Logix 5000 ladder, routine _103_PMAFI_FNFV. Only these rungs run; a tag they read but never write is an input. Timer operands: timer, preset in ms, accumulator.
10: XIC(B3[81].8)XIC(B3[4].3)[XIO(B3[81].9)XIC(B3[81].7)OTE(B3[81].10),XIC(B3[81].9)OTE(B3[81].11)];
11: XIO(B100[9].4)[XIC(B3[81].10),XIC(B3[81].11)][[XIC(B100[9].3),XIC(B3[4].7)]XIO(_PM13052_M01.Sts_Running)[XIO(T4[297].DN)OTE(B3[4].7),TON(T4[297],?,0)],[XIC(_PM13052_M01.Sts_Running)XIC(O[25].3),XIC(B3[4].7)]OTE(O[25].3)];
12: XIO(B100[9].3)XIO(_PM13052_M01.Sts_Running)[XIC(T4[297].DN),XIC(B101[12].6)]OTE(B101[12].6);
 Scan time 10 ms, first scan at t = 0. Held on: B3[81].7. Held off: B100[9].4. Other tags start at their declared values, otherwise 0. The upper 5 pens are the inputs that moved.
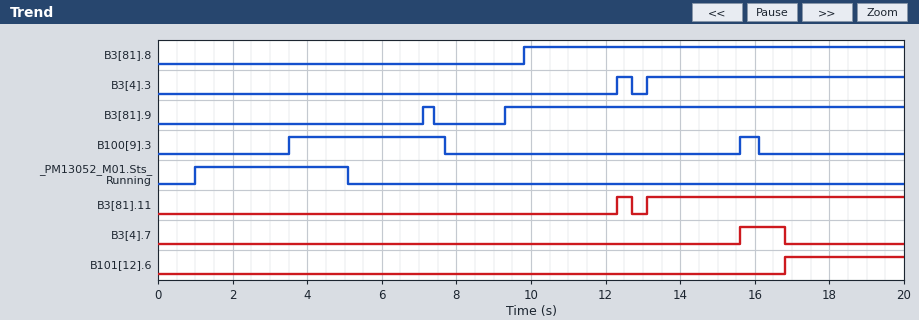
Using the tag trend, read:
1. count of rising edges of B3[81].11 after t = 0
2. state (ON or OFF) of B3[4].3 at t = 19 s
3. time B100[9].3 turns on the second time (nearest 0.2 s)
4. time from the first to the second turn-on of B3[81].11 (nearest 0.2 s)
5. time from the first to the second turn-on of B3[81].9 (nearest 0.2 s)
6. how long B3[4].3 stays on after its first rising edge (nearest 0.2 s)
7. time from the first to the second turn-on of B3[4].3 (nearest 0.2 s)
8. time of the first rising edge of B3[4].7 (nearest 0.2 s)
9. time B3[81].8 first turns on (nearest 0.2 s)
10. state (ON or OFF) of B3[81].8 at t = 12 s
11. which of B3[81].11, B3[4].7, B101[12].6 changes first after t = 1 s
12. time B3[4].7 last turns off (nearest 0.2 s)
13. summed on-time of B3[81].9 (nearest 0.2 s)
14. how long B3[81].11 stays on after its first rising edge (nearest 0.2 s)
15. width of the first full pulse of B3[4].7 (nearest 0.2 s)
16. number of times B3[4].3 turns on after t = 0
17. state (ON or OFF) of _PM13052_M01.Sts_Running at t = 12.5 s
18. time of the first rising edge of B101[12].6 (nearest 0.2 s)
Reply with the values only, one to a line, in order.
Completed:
2
ON
15.6 s
0.8 s
2.2 s
0.4 s
0.8 s
15.6 s
9.8 s
ON
B3[81].11
16.8 s
11.0 s
0.4 s
1.2 s
2
OFF
16.8 s
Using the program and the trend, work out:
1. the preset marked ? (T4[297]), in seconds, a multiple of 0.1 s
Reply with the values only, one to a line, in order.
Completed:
1.2 s
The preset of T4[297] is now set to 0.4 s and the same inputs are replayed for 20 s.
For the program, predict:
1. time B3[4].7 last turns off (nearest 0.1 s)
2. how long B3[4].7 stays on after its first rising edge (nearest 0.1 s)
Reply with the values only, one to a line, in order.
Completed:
16.0 s
0.4 s
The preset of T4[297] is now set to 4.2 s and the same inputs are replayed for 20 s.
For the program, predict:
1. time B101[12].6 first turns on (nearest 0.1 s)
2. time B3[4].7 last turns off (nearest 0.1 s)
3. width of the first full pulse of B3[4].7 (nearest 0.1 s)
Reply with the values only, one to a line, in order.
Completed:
19.8 s
19.8 s
4.2 s
